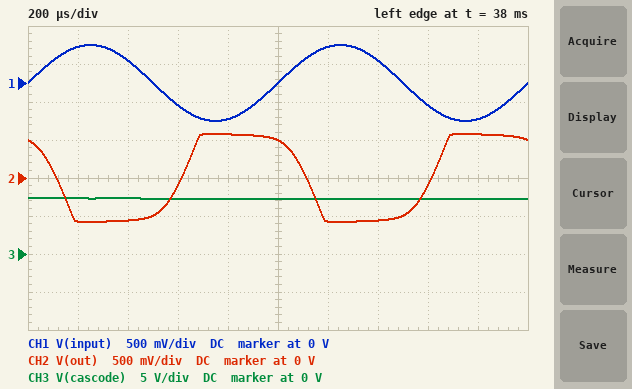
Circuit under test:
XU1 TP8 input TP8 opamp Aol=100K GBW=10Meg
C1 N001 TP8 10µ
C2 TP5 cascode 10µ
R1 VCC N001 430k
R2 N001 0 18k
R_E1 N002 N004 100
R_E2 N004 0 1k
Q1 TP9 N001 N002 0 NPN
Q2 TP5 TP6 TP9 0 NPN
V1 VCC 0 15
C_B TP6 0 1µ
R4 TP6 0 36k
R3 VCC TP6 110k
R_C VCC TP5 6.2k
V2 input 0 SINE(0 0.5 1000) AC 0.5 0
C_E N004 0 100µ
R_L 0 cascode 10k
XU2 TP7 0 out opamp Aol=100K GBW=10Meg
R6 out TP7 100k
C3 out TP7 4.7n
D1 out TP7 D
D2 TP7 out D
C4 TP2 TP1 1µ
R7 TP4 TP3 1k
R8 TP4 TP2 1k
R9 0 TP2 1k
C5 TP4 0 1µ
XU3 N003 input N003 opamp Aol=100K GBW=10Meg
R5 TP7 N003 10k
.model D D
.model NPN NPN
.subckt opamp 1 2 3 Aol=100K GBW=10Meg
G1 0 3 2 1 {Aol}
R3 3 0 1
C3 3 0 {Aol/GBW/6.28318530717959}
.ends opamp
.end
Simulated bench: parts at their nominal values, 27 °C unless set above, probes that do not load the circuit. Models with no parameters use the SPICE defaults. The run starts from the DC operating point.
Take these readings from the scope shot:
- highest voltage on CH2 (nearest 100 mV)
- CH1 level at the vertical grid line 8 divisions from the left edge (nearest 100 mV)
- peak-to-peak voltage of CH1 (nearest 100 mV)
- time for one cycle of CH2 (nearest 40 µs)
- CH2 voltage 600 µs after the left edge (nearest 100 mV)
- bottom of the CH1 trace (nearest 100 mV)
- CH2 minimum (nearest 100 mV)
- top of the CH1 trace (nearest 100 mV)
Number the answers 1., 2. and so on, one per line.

1. 600 mV
2. -300 mV
3. 1.0 V
4. 1.00 ms
5. -100 mV
6. -500 mV
7. -600 mV
8. 500 mV
